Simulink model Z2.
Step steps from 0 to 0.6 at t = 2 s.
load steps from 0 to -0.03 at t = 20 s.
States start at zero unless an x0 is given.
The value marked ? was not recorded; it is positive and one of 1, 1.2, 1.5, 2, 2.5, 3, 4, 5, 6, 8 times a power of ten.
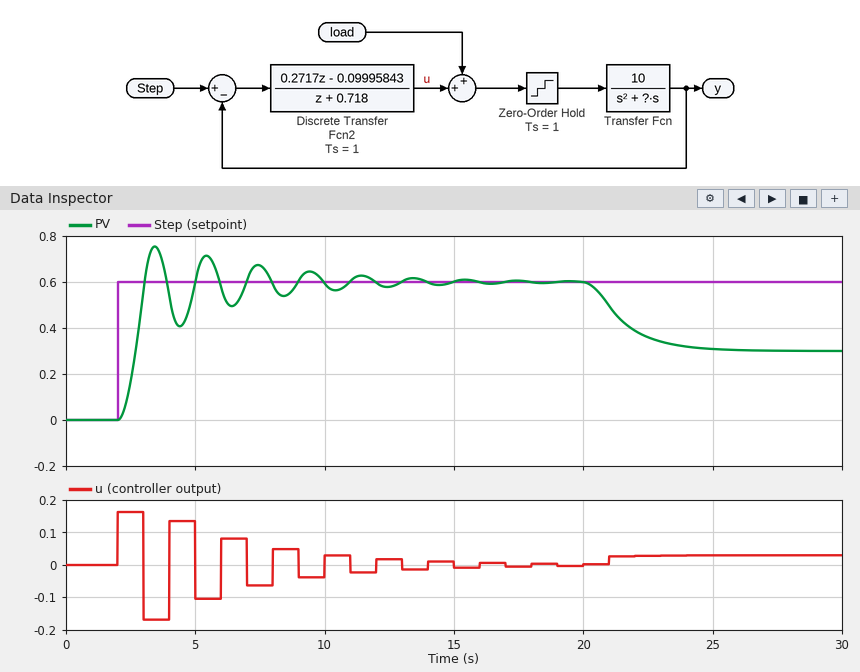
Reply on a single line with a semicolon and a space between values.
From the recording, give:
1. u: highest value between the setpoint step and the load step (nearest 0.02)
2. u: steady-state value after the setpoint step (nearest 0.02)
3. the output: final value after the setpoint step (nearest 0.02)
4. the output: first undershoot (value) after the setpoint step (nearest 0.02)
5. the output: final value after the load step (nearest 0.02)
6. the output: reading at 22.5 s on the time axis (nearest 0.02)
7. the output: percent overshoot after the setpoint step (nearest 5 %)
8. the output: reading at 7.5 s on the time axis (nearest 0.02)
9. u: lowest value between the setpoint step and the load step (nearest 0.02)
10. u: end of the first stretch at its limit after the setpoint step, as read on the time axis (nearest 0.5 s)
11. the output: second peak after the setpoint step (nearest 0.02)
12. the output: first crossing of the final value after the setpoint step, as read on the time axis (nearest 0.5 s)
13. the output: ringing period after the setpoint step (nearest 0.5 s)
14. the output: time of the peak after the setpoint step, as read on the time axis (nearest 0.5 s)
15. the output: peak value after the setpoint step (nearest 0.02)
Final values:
0.16; 0.00; 0.60; 0.40; 0.30; 0.36; 25 %; 0.68; -0.16; 3.0 s; 0.72; 3.0 s; 2.0 s; 3.5 s; 0.76
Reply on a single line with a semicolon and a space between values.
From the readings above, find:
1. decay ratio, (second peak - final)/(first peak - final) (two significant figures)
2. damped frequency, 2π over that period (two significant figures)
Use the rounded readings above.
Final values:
0.75; 3.1 rad/s
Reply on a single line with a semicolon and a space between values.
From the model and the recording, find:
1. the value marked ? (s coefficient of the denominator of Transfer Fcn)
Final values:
1.2
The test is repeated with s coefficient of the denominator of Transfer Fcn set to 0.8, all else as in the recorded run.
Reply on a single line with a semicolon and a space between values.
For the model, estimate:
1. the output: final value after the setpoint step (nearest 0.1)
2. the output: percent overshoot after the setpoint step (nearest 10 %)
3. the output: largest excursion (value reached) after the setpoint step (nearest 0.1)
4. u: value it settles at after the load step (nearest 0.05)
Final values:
0.6; 50 %; 0.9; 0.05
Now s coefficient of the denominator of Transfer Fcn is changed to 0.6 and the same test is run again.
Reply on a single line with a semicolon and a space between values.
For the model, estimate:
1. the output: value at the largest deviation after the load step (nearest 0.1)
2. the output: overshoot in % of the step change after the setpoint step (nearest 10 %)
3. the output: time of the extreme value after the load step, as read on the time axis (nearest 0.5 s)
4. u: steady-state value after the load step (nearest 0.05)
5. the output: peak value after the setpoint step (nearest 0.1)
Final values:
0.3; 60 %; 23.0 s; 0.05; 1.0
